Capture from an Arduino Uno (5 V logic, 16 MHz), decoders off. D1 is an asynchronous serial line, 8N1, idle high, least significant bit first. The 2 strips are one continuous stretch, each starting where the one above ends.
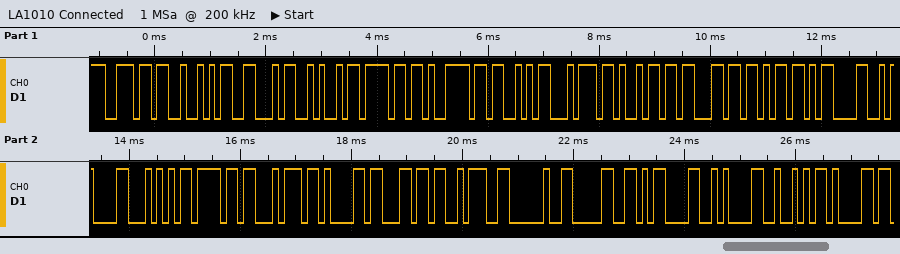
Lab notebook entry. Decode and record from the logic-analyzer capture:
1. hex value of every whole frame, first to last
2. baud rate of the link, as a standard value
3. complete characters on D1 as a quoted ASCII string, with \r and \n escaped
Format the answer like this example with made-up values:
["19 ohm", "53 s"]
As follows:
["0x6E 0x52 0x46 0x4A 0x6F 0x79 0x53 0x74 0x69 0x63 0x6B 0x0D 0x0A 0x54 0x6F 0x74 0x61 0x6C 0x3A 0x20 0x30 0x0D 0x0A 0x52 0x61", "9600 baud", "\"nRFJoyStick\\r\\nTotal: 0\\r\\nRa\""]
